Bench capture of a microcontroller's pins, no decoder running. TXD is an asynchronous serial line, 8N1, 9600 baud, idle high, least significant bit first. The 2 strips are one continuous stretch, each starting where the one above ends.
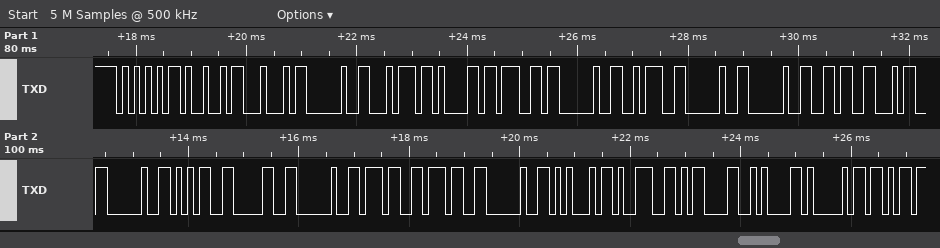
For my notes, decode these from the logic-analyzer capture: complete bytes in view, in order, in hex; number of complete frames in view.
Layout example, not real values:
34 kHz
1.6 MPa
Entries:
55 49 44 20 74 61 67 20 3A 20 20 36 34 20 35 30 20 37 37 20 45 39 0D 0A 41 6B
26
